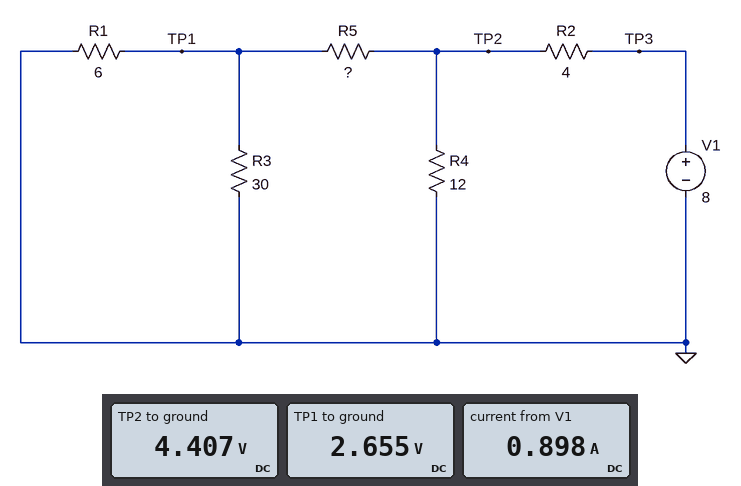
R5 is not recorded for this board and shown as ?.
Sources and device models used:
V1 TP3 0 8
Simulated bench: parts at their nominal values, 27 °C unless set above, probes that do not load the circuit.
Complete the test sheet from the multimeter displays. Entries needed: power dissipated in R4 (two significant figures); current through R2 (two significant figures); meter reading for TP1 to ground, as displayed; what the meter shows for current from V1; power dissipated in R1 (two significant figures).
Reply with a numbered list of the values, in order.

1. 1.6 W
2. 900 mA
3. 2.655 V
4. 0.898 A
5. 1.2 W
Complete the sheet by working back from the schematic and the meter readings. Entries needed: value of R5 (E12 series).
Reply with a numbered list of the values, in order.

1. 3.3 Ω
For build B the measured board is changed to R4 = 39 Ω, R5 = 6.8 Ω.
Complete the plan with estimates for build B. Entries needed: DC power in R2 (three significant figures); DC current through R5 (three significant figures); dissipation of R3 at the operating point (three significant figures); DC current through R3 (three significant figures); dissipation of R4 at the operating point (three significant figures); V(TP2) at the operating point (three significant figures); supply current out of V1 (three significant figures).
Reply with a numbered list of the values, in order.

1. 1.50 W
2. 470 mA
3. 184 mW
4. 78.4 mA
5. 790 mW
6. 5.55 V
7. 613 mA
